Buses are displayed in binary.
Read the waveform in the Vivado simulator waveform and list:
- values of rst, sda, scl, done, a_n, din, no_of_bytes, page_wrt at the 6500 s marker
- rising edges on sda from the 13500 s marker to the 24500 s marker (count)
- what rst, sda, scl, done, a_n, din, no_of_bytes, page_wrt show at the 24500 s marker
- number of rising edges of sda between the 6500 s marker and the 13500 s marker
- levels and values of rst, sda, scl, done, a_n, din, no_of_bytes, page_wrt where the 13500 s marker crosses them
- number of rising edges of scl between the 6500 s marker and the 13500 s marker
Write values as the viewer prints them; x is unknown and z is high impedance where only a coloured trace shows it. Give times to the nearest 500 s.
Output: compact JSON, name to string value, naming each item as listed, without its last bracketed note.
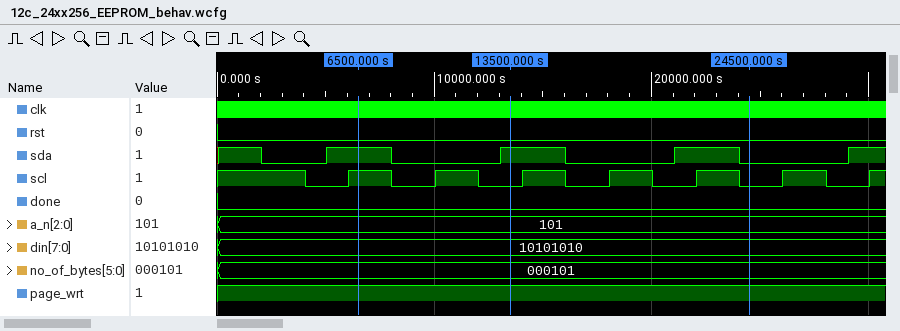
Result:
{"values of rst, sda, scl, done, a_n, din, no_of_bytes, page_wrt at the 6500 s marker": "rst=0, sda=1, scl=1, done=0, a_n=101, din=10101010, no_of_bytes=000101, page_wrt=1", "rising edges on sda from the 13500 s marker to the 24500 s marker": "1", "what rst, sda, scl, done, a_n, din, no_of_bytes, page_wrt show at the 24500 s marker": "rst=0, sda=0, scl=0, done=0, a_n=101, din=10101010, no_of_bytes=000101, page_wrt=1", "number of rising edges of sda between the 6500 s marker and the 13500 s marker": "1", "levels and values of rst, sda, scl, done, a_n, din, no_of_bytes, page_wrt where the 13500 s marker crosses them": "rst=0, sda=1, scl=0, done=0, a_n=101, din=10101010, no_of_bytes=000101, page_wrt=1", "number of rising edges of scl between the 6500 s marker and the 13500 s marker": "1"}
